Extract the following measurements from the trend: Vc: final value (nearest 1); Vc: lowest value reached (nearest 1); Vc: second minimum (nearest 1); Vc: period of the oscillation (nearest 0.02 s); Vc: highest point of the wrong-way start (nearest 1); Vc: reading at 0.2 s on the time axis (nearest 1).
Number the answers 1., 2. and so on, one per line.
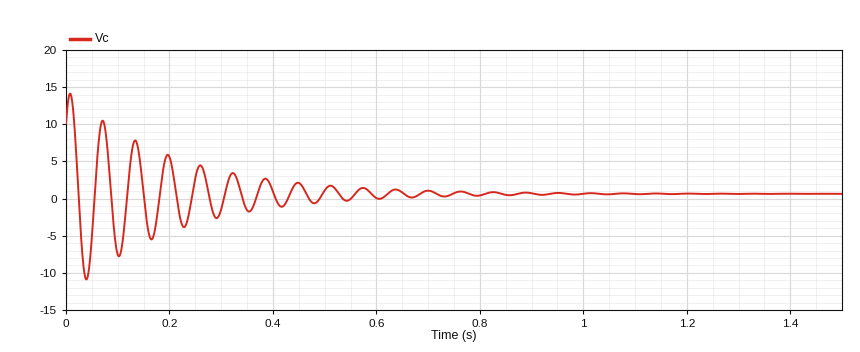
1. 1
2. -11
3. -8
4. 0.06 s
5. 14
6. 6
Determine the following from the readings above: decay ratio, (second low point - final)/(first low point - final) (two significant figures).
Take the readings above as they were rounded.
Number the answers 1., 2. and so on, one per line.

1. 0.75
